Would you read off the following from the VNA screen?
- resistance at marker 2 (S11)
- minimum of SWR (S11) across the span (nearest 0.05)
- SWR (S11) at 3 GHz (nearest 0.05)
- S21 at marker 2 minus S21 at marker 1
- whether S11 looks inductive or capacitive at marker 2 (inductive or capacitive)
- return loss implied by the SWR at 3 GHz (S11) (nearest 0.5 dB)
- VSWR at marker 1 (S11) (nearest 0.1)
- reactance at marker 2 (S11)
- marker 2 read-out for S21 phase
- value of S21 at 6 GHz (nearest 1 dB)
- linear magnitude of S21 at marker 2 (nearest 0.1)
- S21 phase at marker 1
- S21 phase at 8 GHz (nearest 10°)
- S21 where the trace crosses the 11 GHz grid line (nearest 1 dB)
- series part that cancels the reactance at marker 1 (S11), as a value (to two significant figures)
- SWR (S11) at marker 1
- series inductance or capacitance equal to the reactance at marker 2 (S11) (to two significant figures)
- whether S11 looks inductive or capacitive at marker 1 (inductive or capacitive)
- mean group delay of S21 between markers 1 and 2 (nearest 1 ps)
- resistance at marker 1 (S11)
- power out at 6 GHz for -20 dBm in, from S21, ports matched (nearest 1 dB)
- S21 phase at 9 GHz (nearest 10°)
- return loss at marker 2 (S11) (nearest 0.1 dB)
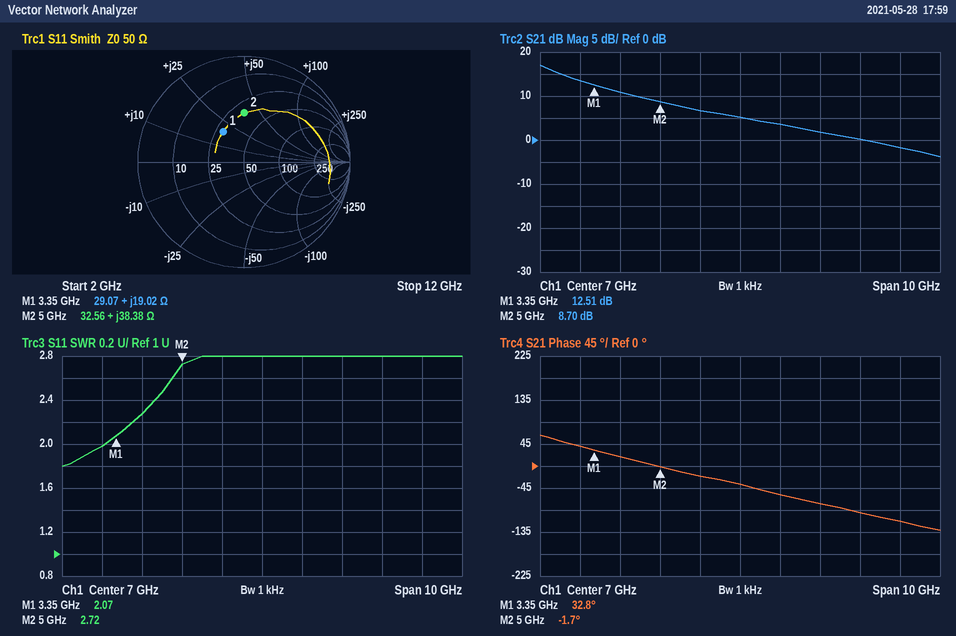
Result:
32.56 Ω
1.80
2.00
-3.81 dB
inductive
9.5 dB
2.1
+38.38 Ω
-1.7°
7 dB
2.7
32.8°
-60°
-2 dB
2.5 pF
2.07
1.2 nH
inductive
58 ps
29.07 Ω
-13 dBm
-80°
6.7 dB
